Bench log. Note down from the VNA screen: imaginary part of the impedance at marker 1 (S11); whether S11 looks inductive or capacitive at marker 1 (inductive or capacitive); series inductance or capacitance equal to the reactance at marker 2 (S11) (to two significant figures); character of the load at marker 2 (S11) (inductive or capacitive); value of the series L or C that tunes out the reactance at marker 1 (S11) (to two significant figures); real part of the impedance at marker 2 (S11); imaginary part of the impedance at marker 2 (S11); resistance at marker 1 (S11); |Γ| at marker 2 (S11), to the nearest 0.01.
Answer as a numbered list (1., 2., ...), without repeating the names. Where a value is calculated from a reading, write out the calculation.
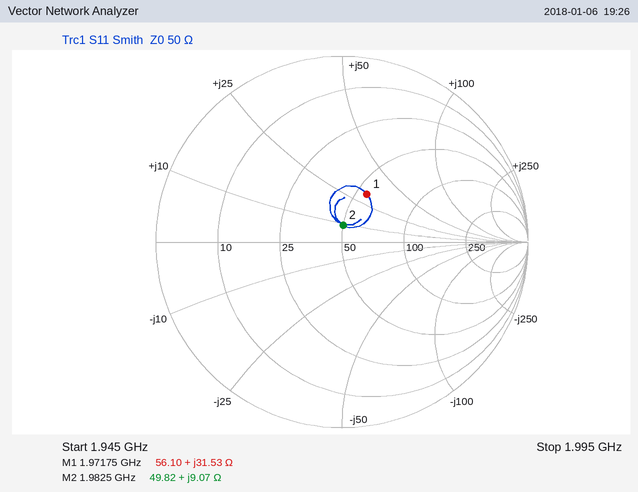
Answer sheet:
1. +31.53 Ω
2. inductive
3. L = 9.07 Ω/(2π × 1.9825 GHz) ≈ 728 pH, so 730 pH to two significant figures
4. inductive
5. C = 1/(2π × 1.97175 GHz × 31.53 Ω) ≈ 2.6 pF
6. 49.82 Ω
7. +9.07 Ω
8. 56.10 Ω
9. 0.09
